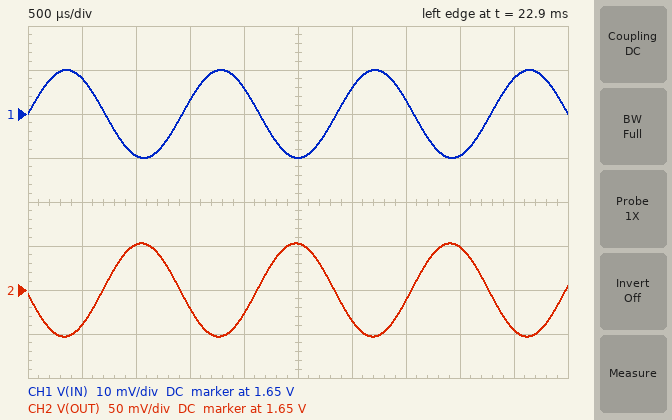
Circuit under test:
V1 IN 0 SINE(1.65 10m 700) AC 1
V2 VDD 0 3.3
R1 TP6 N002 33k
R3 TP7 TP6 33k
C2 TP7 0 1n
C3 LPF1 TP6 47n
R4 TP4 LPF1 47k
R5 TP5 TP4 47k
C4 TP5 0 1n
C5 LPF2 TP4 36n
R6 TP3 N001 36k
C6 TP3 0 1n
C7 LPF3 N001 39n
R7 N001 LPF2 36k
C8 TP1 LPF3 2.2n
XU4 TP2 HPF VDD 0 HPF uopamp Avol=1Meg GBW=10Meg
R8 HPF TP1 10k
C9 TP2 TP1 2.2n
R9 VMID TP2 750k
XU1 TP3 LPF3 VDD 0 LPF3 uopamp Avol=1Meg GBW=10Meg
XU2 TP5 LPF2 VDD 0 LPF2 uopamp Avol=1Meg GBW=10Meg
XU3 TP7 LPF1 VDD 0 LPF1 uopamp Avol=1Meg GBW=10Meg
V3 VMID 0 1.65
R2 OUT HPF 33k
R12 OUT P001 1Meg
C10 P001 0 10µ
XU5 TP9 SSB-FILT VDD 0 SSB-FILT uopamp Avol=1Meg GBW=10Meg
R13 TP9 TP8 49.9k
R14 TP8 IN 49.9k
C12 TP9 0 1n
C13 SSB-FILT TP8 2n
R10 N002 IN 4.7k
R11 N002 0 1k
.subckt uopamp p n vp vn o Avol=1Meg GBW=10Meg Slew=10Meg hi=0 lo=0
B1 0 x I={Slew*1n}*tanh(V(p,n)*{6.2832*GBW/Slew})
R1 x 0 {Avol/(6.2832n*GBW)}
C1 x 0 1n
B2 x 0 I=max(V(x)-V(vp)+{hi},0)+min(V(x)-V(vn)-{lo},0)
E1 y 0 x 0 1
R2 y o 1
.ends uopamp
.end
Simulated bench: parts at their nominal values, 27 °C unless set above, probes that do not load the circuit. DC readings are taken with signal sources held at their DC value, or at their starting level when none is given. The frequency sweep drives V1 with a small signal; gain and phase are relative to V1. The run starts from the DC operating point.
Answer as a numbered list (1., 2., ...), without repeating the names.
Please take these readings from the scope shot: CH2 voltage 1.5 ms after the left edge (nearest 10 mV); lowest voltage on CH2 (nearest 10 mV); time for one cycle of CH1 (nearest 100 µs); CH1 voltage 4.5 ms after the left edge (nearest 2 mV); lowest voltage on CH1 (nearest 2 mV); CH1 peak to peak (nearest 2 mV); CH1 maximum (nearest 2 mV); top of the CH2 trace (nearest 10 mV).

1. 1.63 V
2. 1.60 V
3. 1.4 ms
4. 1.658 V
5. 1.640 V
6. 20 mV
7. 1.660 V
8. 1.70 V
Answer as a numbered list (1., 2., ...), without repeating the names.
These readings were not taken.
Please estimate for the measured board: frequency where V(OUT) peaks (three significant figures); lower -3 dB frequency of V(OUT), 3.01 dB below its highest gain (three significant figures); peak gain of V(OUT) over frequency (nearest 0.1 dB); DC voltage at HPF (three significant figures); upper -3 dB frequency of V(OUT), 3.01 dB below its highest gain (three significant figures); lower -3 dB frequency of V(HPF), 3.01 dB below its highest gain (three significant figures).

1. 692 Hz
2. 617 Hz
3. 14.5 dB
4. 1.65 V
5. 766 Hz
6. 617 Hz
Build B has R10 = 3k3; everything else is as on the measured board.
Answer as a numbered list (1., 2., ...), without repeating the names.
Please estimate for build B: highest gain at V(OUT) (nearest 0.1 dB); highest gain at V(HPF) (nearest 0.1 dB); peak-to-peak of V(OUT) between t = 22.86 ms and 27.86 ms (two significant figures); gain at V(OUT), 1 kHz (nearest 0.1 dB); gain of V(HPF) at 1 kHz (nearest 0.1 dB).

1. 17.0 dB
2. 17.3 dB
3. 140 mV
4. -13.0 dB
5. -12.7 dB
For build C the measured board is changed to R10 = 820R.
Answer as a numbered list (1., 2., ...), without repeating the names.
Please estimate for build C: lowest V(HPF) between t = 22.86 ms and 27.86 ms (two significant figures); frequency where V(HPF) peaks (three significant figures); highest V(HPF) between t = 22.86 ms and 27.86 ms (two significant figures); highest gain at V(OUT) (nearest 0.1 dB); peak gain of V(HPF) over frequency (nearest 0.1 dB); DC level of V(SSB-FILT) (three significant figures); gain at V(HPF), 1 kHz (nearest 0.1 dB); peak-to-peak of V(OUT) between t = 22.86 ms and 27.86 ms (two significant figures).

1. 1.5 V
2. 694 Hz
3. 1.8 V
4. 24.5 dB
5. 24.8 dB
6. 1.65 V
7. -5.1 dB
8. 330 mV
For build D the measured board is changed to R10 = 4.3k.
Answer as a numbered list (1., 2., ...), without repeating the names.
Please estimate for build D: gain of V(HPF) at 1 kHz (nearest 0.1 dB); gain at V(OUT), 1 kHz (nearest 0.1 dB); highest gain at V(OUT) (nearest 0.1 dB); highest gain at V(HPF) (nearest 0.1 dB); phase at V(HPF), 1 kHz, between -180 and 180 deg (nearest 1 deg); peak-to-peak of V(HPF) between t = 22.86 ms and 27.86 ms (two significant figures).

1. -14.5 dB
2. -14.8 dB
3. 15.2 dB
4. 15.4 dB
5. -86 deg
6. 120 mV
